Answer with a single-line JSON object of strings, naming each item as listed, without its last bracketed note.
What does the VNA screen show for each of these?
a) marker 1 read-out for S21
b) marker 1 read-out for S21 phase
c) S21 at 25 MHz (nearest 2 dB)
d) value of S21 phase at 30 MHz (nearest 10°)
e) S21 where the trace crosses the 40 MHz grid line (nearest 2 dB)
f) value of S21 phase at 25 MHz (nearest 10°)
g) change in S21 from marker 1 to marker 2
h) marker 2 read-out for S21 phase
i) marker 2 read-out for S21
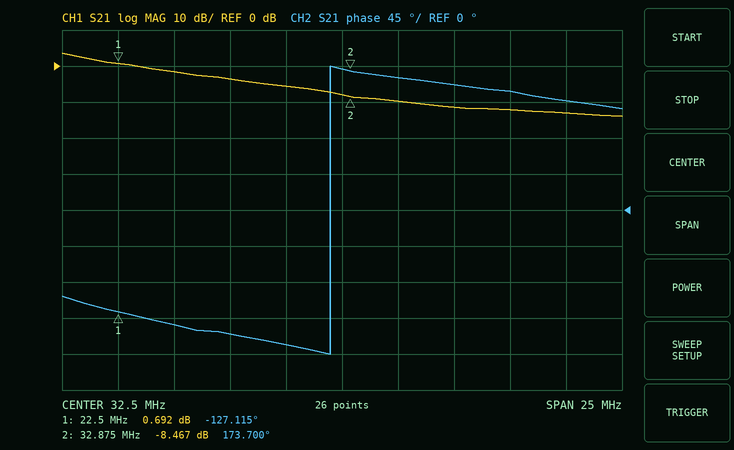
{"marker 1 read-out for S21": "0.692 dB", "marker 1 read-out for S21 phase": "-127.115°", "S21 at 25 MHz": "-2 dB", "value of S21 phase at 30 MHz": "-170°", "S21 where the trace crosses the 40 MHz grid line": "-12 dB", "value of S21 phase at 25 MHz": "-140°", "change in S21 from marker 1 to marker 2": "-9.159 dB", "marker 2 read-out for S21 phase": "173.700°", "marker 2 read-out for S21": "-8.467 dB"}
